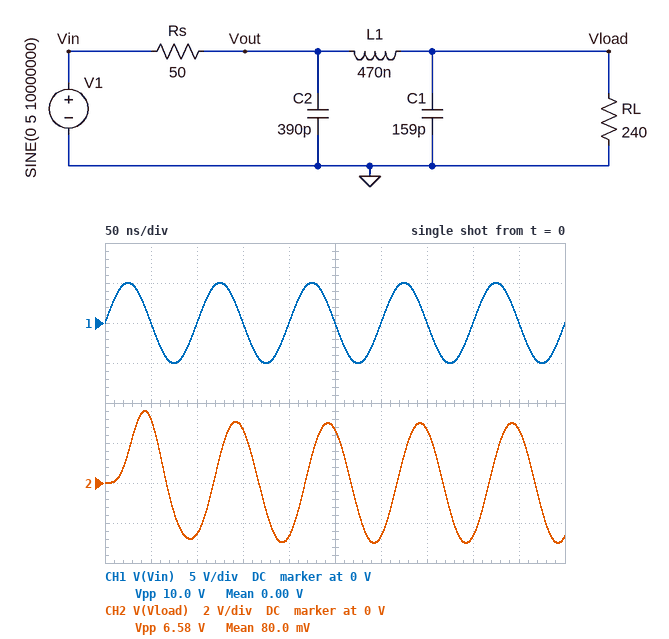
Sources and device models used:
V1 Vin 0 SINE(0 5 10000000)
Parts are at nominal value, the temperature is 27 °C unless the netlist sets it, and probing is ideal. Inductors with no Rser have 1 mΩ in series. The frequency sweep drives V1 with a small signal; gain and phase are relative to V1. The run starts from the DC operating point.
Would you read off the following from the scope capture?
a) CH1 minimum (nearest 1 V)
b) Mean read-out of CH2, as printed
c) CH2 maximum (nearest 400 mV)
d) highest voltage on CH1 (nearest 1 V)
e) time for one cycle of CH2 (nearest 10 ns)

-5 V
80.0 mV
3.6 V
5 V
100 ns
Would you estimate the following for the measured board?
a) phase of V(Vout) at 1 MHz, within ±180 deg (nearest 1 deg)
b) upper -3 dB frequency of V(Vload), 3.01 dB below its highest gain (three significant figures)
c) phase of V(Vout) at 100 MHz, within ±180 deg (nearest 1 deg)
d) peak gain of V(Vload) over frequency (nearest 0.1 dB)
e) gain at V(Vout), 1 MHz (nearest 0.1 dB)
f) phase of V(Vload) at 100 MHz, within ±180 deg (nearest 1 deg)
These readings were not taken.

-8 deg
23.5 MHz
-85 deg
0.7 dB
-1.7 dB
97 deg
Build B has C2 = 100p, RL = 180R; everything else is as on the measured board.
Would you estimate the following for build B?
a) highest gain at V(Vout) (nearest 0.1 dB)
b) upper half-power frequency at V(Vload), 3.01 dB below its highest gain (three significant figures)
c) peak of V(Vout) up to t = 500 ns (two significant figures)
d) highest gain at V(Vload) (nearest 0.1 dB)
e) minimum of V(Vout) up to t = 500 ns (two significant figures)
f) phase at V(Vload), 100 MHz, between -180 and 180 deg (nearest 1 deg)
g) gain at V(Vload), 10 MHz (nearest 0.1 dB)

-0.7 dB
28.9 MHz
2.8 V
-1.7 dB
-2.8 V
112 deg
-2.2 dB
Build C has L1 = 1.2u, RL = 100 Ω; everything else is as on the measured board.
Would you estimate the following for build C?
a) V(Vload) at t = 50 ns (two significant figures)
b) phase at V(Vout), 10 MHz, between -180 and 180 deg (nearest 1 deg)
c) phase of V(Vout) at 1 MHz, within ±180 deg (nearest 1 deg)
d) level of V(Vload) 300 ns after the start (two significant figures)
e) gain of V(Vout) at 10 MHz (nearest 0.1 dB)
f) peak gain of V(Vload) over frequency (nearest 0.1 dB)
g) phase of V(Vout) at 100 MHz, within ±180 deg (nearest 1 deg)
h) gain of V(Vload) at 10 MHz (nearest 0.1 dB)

2.7 V
-25 deg
-5 deg
-3.2 V
-5.9 dB
-3.5 dB
-85 deg
-3.9 dB
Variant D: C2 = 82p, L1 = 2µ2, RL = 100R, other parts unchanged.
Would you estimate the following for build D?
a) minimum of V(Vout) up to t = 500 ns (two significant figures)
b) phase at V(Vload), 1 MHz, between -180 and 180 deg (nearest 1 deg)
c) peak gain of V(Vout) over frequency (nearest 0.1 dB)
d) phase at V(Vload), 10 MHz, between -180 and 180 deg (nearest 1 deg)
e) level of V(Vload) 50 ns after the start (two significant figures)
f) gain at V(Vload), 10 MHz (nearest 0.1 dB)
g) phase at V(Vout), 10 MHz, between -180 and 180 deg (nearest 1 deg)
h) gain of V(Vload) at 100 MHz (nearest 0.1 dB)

-4.0 V
-8 deg
-0.4 dB
-98 deg
2.6 V
-5.1 dB
8 deg
-51.5 dB
